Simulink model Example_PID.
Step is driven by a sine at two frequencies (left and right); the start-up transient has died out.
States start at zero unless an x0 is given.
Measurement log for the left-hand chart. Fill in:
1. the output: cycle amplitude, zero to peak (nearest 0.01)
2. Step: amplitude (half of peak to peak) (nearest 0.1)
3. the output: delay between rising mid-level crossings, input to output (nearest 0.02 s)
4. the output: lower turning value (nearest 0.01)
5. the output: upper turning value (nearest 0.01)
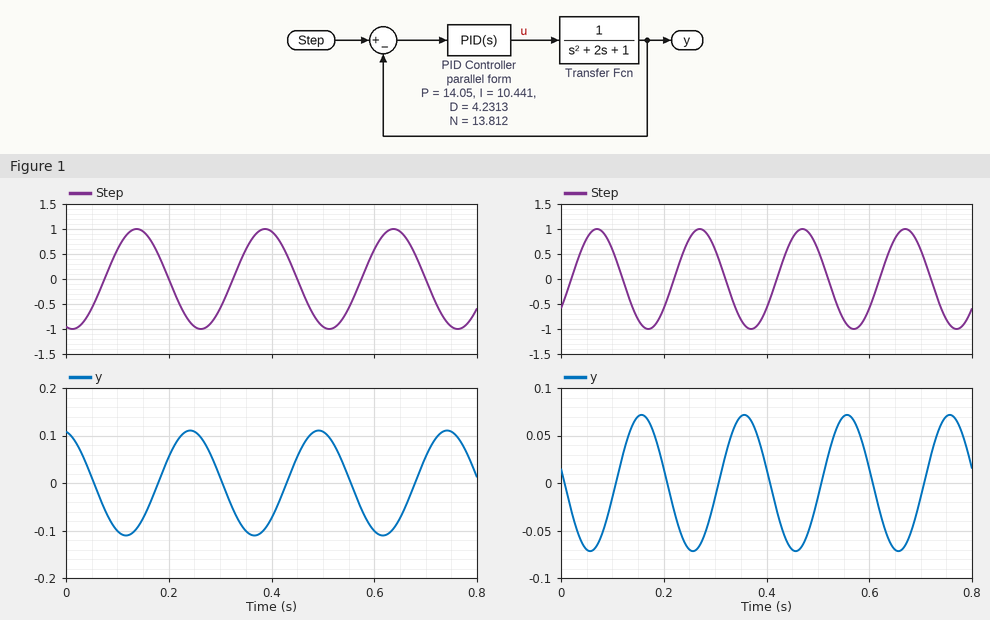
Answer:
0.11
1.0
0.10 s
-0.11
0.11
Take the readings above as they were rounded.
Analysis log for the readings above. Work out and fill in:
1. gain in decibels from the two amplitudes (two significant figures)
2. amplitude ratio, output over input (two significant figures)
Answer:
-19 dB
0.11
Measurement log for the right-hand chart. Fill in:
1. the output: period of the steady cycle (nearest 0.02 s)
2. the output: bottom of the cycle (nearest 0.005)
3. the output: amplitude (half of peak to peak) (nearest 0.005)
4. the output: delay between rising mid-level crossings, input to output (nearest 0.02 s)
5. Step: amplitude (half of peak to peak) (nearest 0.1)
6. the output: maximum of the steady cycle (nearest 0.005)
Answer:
0.20 s
-0.070
0.070
0.08 s
1.0
0.070
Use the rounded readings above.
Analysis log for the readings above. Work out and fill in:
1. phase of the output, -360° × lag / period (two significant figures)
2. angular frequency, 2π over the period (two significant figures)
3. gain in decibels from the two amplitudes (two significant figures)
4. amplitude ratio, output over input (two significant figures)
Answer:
-140°
31 rad/s
-23 dB
0.070
